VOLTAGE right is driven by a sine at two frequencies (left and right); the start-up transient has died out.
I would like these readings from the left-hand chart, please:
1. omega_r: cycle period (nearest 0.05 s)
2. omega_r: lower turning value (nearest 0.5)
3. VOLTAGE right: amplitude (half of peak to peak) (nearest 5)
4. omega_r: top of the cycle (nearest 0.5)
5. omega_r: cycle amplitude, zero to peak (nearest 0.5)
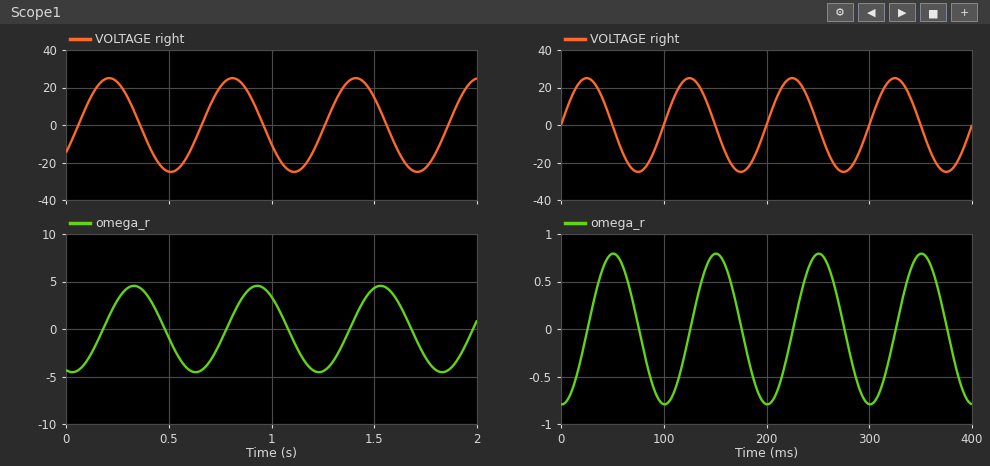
0.60 s
-4.5
25
4.5
4.5
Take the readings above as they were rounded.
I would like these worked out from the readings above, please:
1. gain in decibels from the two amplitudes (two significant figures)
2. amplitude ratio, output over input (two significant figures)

-15 dB
0.18
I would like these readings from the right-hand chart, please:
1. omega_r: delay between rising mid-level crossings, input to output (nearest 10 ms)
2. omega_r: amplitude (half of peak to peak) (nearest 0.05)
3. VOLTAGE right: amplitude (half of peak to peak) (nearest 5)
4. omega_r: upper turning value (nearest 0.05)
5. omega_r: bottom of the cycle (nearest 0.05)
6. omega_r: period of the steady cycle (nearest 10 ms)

30 ms
0.80
25
0.80
-0.80
100 ms
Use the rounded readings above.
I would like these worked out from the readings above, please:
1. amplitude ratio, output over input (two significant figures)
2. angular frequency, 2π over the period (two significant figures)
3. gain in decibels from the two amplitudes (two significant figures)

0.032
0.063 rad/ms
-30 dB
